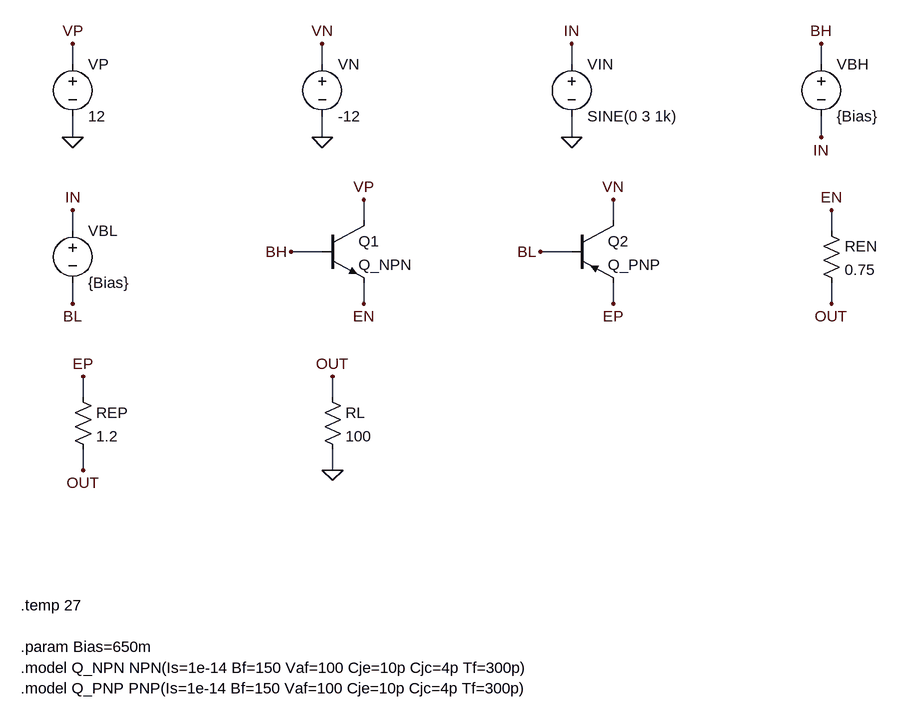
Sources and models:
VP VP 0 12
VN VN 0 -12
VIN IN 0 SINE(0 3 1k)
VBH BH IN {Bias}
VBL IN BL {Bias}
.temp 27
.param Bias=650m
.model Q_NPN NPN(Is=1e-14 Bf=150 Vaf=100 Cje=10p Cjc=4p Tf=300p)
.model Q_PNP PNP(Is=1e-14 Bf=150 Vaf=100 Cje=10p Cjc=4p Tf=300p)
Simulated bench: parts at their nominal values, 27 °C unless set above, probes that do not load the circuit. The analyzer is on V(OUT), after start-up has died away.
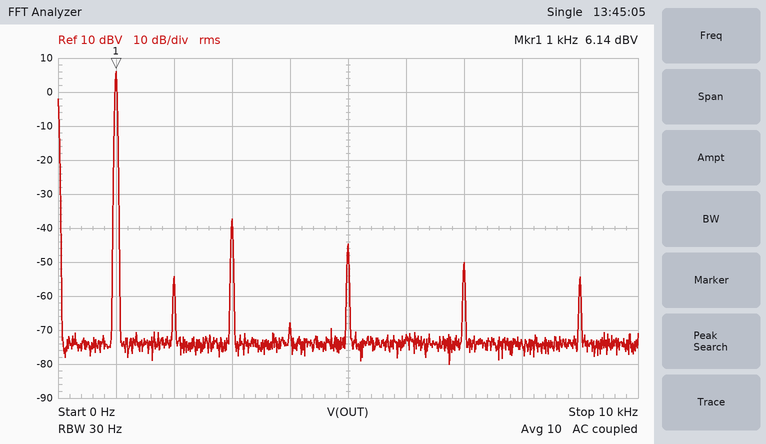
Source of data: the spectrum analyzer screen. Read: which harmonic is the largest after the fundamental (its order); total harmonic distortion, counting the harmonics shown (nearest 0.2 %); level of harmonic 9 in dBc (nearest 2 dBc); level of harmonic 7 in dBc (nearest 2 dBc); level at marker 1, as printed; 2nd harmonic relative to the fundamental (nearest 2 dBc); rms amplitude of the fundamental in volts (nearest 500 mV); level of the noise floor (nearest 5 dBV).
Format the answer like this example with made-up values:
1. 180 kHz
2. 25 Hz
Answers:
1. 3
2. 0.8 %
3. -60 dBc
4. -56 dBc
5. 6.14 dBV
6. -60 dBc
7. 2.0 V
8. -75 dBV
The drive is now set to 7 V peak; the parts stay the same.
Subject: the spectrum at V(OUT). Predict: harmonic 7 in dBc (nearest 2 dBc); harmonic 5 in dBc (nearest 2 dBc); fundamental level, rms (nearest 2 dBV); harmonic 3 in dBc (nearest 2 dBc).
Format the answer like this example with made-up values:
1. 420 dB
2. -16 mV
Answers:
1. -58 dBc
2. -54 dBc
3. 14 dBV
4. -48 dBc
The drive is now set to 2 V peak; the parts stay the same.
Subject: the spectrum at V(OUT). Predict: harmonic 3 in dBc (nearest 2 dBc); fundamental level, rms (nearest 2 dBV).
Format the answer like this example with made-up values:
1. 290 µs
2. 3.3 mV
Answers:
1. -42 dBc
2. 2 dBV
